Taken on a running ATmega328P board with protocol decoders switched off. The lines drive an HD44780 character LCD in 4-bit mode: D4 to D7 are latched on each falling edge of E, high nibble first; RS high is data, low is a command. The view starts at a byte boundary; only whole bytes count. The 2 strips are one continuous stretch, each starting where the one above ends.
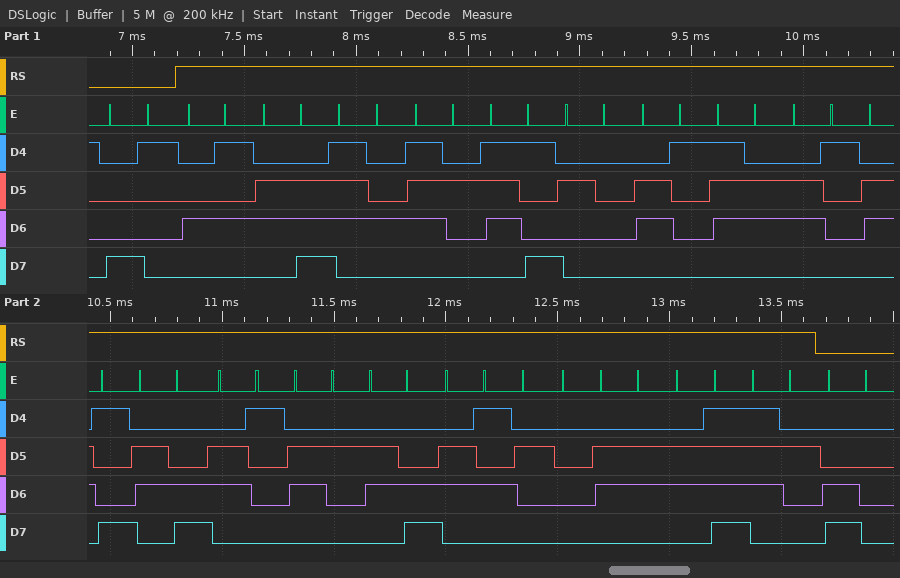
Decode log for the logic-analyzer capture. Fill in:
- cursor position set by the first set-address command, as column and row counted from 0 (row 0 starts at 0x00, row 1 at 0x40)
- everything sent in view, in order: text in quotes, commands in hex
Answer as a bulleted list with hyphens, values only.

- column 1, row 0
- 0x81 "Entry available for" 0xC0
